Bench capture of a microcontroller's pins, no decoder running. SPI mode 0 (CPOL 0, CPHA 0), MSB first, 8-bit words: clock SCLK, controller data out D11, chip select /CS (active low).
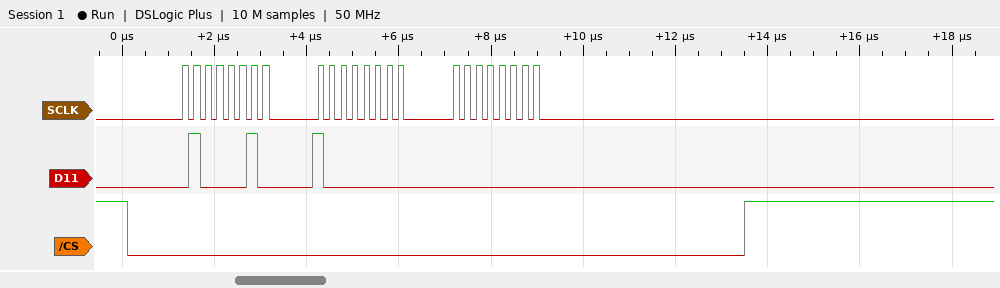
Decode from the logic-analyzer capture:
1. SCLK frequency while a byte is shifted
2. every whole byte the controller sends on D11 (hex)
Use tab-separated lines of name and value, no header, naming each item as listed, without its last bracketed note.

SCLK frequency while a byte is shifted	4 MHz
every whole byte the controller sends on D11	0x42 0x80 0x00
